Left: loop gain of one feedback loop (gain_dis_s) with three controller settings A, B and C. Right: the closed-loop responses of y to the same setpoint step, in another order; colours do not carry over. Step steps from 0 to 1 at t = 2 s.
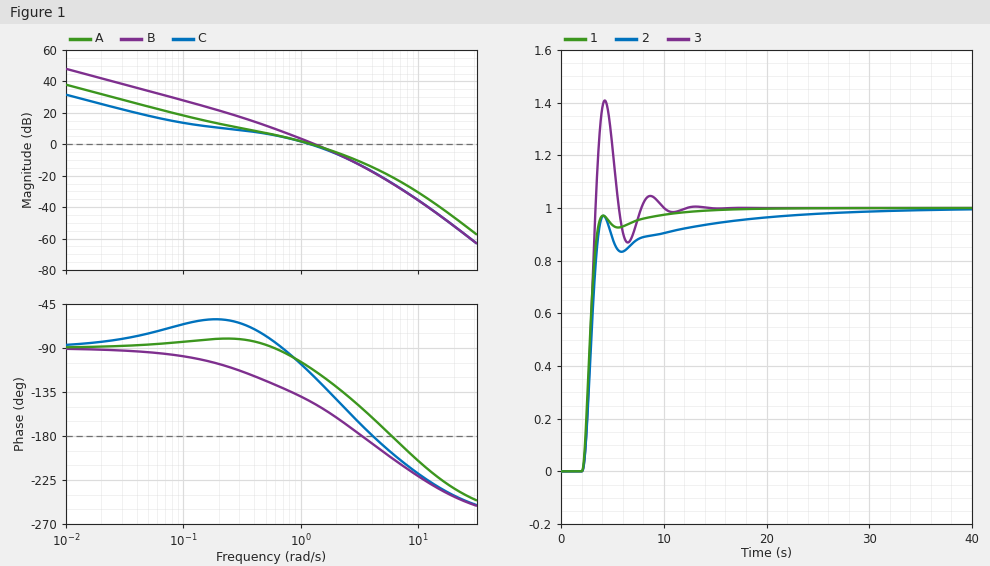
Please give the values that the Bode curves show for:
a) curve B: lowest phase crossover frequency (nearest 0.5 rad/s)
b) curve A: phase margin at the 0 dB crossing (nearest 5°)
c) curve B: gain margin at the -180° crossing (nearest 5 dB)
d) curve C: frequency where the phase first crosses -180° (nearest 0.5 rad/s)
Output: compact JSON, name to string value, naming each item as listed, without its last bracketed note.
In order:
{"curve B: lowest phase crossover frequency": "3.5 rad/s", "curve A: phase margin at the 0 dB crossing": "70°", "curve B: gain margin at the -180° crossing": "15 dB", "curve C: frequency where the phase first crosses -180°": "4.0 rad/s"}
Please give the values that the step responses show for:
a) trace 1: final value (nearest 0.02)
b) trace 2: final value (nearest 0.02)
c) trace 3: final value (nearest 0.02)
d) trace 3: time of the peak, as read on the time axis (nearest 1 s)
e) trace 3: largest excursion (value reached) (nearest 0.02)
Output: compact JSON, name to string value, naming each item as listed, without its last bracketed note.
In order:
{"trace 1: final value": "1.00", "trace 2: final value": "1.00", "trace 3: final value": "1.00", "trace 3: time of the peak, as read on the time axis": "4 s", "trace 3: largest excursion (value reached)": "1.40"}
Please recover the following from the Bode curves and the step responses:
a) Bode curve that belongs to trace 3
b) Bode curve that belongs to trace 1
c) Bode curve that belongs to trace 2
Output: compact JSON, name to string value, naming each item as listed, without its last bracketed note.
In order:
{"Bode curve that belongs to trace 3": "B", "Bode curve that belongs to trace 1": "A", "Bode curve that belongs to trace 2": "C"}
